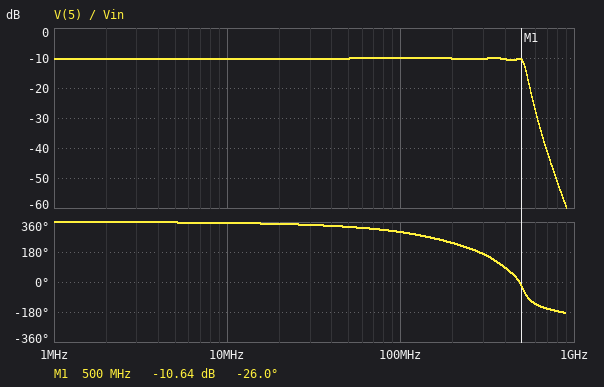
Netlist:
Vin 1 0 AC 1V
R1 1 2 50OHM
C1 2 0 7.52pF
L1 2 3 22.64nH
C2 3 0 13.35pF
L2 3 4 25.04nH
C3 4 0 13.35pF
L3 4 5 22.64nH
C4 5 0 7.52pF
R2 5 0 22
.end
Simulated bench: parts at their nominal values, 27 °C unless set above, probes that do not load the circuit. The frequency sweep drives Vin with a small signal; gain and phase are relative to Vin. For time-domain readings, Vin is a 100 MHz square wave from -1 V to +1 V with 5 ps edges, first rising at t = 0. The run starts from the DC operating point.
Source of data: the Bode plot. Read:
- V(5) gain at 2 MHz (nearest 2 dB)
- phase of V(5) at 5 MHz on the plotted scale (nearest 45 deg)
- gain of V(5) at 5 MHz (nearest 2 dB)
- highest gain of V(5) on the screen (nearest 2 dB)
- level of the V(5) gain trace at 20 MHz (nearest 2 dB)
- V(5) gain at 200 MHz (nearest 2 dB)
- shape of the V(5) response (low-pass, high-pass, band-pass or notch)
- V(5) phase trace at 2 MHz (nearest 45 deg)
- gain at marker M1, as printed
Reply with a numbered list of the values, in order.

1. -10 dB
2. 360 deg
3. -10 dB
4. -10 dB
5. -10 dB
6. -10 dB
7. low-pass
8. 360 deg
9. -10.64 dB
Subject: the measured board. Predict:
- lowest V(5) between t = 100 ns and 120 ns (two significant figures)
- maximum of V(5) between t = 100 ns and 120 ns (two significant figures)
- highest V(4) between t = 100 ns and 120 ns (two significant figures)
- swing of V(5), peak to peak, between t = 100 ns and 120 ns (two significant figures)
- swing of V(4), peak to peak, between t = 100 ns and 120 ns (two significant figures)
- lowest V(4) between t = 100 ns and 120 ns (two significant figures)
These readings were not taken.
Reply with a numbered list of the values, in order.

1. -450 mV
2. 450 mV
3. 840 mV
4. 900 mV
5. 1.7 V
6. -840 mV
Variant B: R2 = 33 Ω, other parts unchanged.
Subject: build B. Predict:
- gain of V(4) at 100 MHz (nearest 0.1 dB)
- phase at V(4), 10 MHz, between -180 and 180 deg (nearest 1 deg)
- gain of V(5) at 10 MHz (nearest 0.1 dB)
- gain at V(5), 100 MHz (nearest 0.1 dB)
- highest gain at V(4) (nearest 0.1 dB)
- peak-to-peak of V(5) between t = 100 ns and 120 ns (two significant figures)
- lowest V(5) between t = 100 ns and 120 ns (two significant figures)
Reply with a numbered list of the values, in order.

1. -7.6 dB
2. -4 deg
3. -8.0 dB
4. -7.9 dB
5. -1.1 dB
6. 1.1 V
7. -570 mV
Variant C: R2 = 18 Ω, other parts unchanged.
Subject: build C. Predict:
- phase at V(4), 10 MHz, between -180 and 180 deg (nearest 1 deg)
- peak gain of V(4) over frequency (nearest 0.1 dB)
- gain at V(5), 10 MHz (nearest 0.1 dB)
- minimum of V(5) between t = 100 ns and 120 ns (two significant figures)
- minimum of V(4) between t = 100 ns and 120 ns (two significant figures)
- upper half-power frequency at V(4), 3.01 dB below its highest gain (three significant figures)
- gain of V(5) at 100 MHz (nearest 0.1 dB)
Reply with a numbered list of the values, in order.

1. -1 deg
2. 0.3 dB
3. -11.5 dB
4. -390 mV
5. -870 mV
6. 525 MHz
7. -11.1 dB
